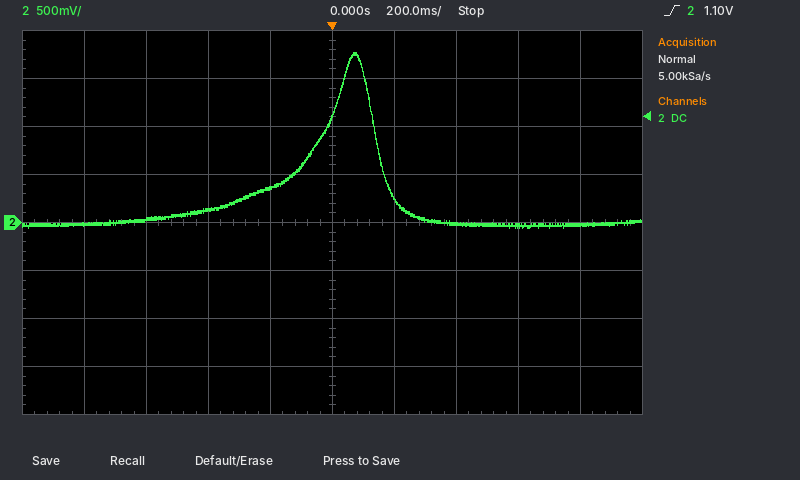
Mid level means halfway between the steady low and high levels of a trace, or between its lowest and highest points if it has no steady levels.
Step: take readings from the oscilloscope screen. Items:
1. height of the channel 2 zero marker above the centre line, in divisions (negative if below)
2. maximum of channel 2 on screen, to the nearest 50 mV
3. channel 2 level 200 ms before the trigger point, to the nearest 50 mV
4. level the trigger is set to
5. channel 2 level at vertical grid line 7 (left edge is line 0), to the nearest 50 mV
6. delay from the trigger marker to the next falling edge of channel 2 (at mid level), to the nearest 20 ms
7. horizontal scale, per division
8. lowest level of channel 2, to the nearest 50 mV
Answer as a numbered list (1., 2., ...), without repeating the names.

1. 0.0 div
2. 1.75 V
3. 350 mV
4. 1.10 V
5. 0 mV
6. 140 ms
7. 200 ms
8. -50 mV
